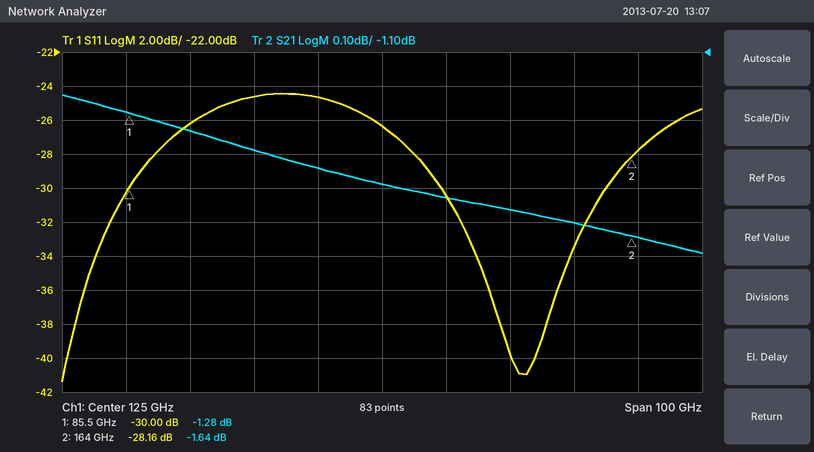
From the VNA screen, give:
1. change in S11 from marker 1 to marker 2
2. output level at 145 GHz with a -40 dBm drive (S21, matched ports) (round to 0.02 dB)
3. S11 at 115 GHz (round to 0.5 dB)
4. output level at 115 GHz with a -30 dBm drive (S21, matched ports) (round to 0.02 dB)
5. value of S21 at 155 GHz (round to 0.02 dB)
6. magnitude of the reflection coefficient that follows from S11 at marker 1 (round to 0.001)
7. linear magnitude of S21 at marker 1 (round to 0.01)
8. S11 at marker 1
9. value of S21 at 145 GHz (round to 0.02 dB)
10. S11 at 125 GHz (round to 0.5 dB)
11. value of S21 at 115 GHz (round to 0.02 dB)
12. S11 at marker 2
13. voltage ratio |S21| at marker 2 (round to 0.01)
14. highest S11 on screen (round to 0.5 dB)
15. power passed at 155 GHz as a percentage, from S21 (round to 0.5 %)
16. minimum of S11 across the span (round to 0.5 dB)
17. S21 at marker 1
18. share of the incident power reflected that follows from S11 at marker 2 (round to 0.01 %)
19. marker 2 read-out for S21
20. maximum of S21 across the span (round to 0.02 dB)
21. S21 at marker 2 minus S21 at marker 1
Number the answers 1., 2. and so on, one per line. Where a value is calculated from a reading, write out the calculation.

1. -28.16 − (-30) = 1.84 dB
2. -40 dBm + (-1.56 dB) = -41.56 dBm
3. -24.5 dB
4. -30 dBm + (-1.44 dB) = -31.44 dBm
5. -1.60 dB
6. 10^(-30/20) ≈ 0.032
7. 10^(-1.28/20) ≈ 0.86
8. -30.00 dB
9. -1.56 dB
10. -26.5 dB
11. -1.44 dB
12. -28.16 dB
13. 10^(-1.64/20) ≈ 0.83
14. -24.5 dB
15. 10^(-1.6/10) ≈ 69.2 %, so 69.0 % to the nearest 0.5 %
16. -41.5 dB
17. -1.28 dB
18. 10^(-28.16/10) ≈ 0.15 %
19. -1.64 dB
20. -1.22 dB
21. -1.64 − (-1.28) = -0.36 dB
